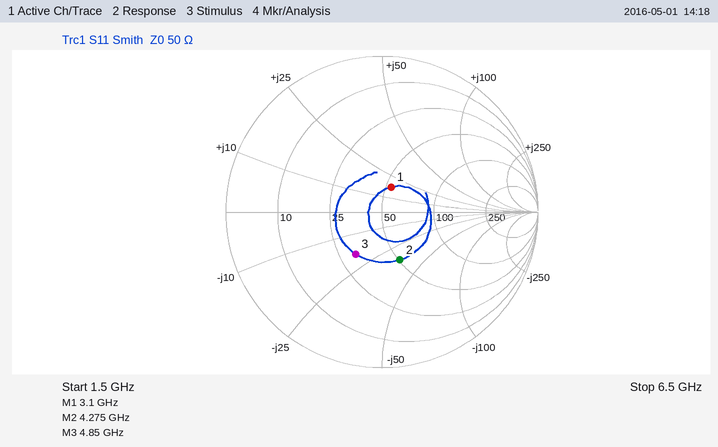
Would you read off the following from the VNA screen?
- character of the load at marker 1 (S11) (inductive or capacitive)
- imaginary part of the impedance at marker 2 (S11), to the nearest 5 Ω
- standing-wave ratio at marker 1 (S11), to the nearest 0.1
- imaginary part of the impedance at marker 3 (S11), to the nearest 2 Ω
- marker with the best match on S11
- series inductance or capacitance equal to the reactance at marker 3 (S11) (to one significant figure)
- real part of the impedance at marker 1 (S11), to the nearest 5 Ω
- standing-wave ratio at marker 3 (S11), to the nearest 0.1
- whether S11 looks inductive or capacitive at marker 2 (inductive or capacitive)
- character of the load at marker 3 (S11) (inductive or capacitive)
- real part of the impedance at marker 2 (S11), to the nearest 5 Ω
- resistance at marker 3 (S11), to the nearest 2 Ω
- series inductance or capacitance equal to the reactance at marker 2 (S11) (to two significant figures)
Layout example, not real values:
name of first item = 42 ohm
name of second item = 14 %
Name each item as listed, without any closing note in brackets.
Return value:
character of the load at marker 1 (S11) = inductive
imaginary part of the impedance at marker 2 (S11), to the nearest 5 Ω = -35 Ω
standing-wave ratio at marker 1 (S11), to the nearest 0.1 = 1.4
imaginary part of the impedance at marker 3 (S11), to the nearest 2 Ω = -18 Ω
marker with the best match on S11 = marker 1
series inductance or capacitance equal to the reactance at marker 3 (S11) = 2 pF
real part of the impedance at marker 1 (S11), to the nearest 5 Ω = 55 Ω
standing-wave ratio at marker 3 (S11), to the nearest 0.1 = 1.9
whether S11 looks inductive or capacitive at marker 2 = capacitive
character of the load at marker 3 (S11) = capacitive
real part of the impedance at marker 2 (S11), to the nearest 5 Ω = 50 Ω
resistance at marker 3 (S11), to the nearest 2 Ω = 32 Ω
series inductance or capacitance equal to the reactance at marker 2 (S11) = 1.1 pF
